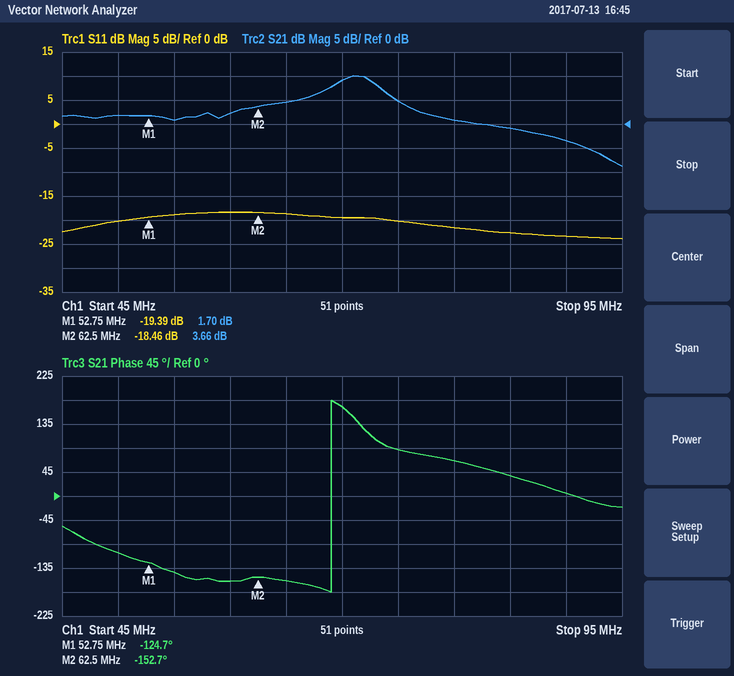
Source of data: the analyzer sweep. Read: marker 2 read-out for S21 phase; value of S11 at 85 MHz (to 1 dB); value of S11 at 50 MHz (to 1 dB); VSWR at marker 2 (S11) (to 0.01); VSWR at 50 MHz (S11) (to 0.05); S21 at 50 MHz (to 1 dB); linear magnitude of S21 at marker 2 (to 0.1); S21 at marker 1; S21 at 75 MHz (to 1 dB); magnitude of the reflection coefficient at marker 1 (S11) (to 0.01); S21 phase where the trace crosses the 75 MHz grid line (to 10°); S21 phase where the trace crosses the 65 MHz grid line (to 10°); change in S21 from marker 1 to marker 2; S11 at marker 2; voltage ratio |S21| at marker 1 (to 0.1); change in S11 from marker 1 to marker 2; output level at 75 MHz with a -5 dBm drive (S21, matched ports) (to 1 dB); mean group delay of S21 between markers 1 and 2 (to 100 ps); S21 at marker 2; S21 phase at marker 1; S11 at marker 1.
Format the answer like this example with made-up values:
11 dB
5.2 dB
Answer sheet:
-152.7°
-23 dB
-20 dB
1.27
1.20
2 dB
1.5
1.70 dB
5 dB
0.11
90°
-160°
1.96 dB
-18.46 dB
1.2
0.93 dB
0 dBm
8.0 ns
3.66 dB
-124.7°
-19.39 dB
